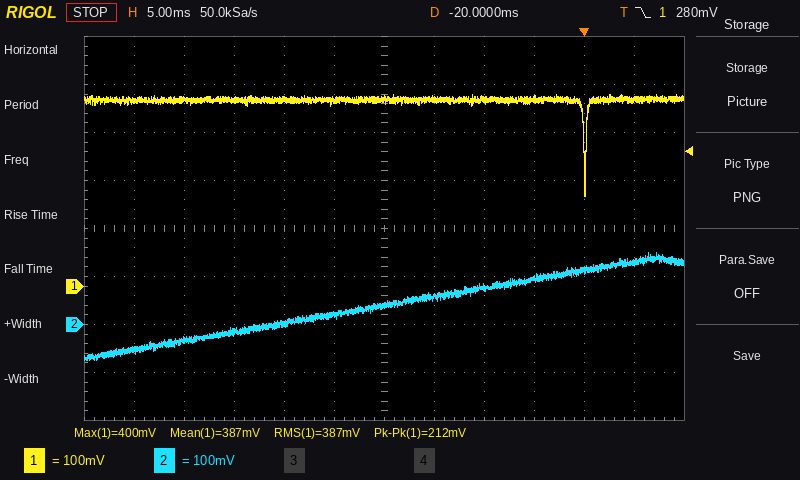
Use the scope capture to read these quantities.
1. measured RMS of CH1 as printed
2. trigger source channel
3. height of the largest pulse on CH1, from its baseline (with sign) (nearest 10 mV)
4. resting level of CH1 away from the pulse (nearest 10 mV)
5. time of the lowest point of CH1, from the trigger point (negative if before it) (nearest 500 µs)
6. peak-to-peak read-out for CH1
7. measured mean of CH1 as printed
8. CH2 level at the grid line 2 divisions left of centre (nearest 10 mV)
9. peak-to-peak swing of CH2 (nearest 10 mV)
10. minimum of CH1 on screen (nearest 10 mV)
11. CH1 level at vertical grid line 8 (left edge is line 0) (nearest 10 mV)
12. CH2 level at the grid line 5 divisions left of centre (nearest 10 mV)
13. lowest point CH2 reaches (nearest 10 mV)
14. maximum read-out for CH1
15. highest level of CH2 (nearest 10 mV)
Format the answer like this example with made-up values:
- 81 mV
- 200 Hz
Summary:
- 387 mV
- CH1
- -200 mV
- 390 mV
- 0.0 ms
- 212 mV
- 387 mV
- 0 mV
- 220 mV
- 190 mV
- 390 mV
- -50 mV
- -70 mV
- 400 mV
- 150 mV
